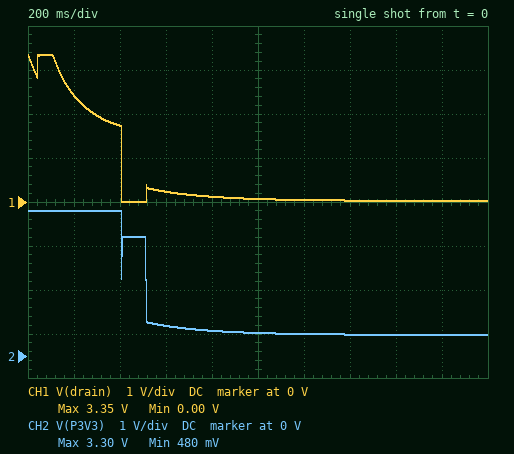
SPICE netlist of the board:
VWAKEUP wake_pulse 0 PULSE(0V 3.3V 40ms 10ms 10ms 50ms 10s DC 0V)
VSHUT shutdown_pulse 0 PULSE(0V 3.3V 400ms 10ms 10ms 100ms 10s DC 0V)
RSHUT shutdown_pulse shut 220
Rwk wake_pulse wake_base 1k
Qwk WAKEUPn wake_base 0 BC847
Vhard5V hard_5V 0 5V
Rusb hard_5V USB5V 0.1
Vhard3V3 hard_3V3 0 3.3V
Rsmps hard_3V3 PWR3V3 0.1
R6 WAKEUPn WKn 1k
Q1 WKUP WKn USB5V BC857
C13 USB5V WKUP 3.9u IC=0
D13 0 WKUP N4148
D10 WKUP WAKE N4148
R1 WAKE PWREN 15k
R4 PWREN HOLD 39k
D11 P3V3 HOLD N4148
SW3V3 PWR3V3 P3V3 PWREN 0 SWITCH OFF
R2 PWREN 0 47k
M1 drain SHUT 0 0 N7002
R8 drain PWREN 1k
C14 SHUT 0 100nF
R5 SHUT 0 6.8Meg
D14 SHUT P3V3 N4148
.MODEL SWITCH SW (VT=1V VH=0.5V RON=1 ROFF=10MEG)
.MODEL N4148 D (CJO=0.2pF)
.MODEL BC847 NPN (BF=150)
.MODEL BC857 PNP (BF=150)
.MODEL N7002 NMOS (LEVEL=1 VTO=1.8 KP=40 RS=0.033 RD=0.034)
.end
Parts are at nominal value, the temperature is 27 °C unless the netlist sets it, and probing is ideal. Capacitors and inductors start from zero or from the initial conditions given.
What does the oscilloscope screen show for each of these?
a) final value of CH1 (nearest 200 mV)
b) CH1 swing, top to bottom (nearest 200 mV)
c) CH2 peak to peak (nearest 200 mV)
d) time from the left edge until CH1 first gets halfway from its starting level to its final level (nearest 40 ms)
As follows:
0 V
3.4 V
2.8 V
400 ms
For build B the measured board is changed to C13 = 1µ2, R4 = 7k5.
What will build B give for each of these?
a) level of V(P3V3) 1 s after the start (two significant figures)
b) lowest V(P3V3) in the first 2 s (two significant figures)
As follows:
470 mV
460 mV
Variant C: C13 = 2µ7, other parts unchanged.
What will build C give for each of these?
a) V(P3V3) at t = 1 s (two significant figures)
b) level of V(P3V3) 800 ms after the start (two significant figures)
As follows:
490 mV
510 mV
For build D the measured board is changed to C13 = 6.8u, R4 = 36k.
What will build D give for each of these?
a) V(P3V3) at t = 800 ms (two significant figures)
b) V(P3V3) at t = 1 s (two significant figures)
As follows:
830 mV
700 mV
